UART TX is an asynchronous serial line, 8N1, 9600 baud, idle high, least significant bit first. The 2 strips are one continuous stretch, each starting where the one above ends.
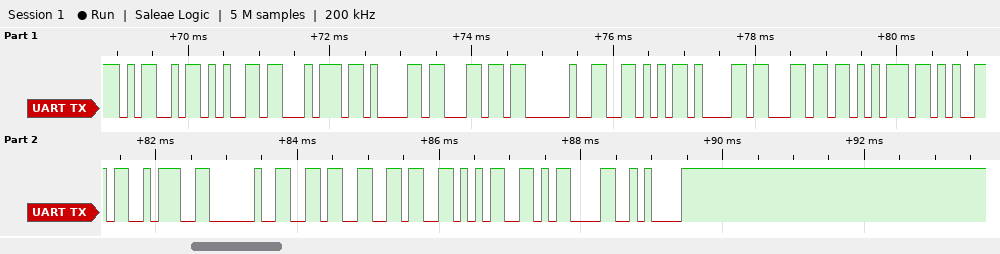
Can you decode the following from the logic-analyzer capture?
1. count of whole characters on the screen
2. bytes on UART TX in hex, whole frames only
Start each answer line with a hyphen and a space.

- 18
- 4D 65 74 61 6C 20 56 61 6C 75 65 3A 20 36 36 35 0D 0A
